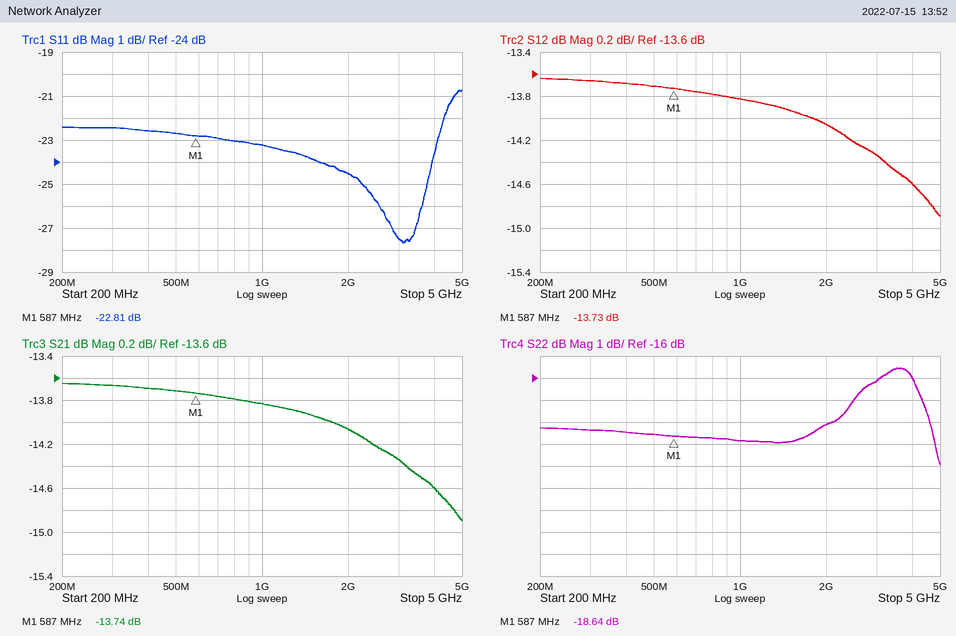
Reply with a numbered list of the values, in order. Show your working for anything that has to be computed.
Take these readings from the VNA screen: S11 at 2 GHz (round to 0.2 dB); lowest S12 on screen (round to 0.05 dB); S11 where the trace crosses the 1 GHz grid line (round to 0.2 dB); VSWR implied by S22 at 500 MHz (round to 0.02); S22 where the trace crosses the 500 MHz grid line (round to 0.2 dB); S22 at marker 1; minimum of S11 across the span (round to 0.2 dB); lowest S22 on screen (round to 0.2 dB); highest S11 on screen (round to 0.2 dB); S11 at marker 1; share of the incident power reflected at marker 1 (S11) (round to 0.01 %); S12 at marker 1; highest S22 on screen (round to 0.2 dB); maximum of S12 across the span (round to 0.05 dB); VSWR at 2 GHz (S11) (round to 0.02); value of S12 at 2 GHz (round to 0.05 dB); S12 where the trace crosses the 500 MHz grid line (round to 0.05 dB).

1. -24.6 dB
2. -14.90 dB
3. -23.2 dB
4. |Γ| = 10^(-18.6/20) = 0.1175; VSWR = (1 + 0.1175)/(1 − 0.1175) ≈ 1.27, so 1.26 to the nearest 0.02
5. -18.6 dB
6. -18.64 dB
7. -27.6 dB
8. -20.0 dB
9. -20.8 dB
10. -22.81 dB
11. 10^(-22.81/10) ≈ 0.52 %
12. -13.73 dB
13. -15.6 dB
14. -13.65 dB
15. |Γ| = 10^(-24.6/20) = 0.0589; VSWR = (1 + 0.0589)/(1 − 0.0589) ≈ 1.13, so 1.12 to the nearest 0.02
16. -14.05 dB
17. -13.70 dB
